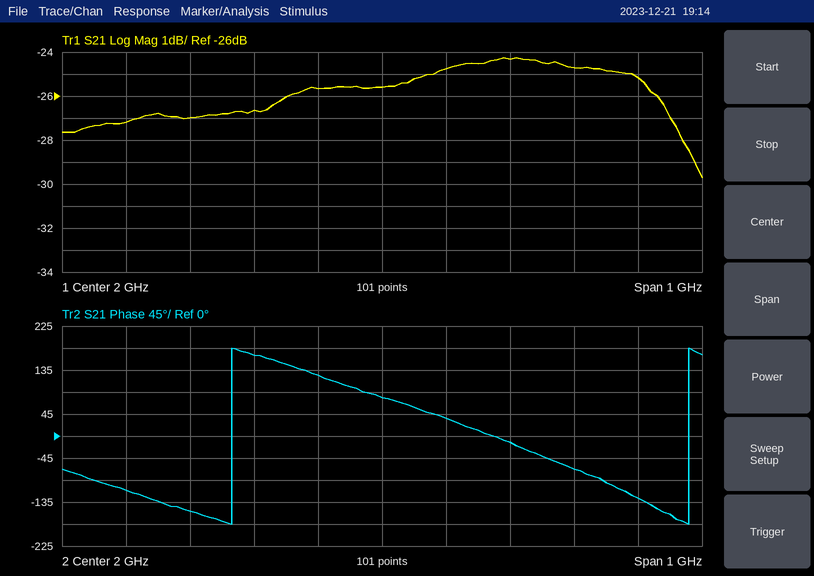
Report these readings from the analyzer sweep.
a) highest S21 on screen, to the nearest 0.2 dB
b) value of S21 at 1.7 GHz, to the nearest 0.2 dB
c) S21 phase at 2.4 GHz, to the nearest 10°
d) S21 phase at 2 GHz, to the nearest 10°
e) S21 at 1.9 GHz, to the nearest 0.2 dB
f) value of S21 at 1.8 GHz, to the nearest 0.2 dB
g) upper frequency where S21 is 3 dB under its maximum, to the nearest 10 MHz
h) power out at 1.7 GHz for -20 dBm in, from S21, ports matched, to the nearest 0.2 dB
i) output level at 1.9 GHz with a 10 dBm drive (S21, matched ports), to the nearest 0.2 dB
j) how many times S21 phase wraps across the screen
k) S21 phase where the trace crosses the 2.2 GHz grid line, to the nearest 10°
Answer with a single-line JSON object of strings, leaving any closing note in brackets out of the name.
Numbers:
{"highest S21 on screen, to the nearest 0.2 dB": "-24.2 dB", "value of S21 at 1.7 GHz, to the nearest 0.2 dB": "-27.0 dB", "S21 phase at 2.4 GHz, to the nearest 10°": "-130°", "S21 phase at 2 GHz, to the nearest 10°": "80°", "S21 at 1.9 GHz, to the nearest 0.2 dB": "-25.6 dB", "value of S21 at 1.8 GHz, to the nearest 0.2 dB": "-26.6 dB", "upper frequency where S21 is 3 dB under its maximum, to the nearest 10 MHz": "2.46 GHz", "power out at 1.7 GHz for -20 dBm in, from S21, ports matched, to the nearest 0.2 dB": "-47.0 dBm", "output level at 1.9 GHz with a 10 dBm drive (S21, matched ports), to the nearest 0.2 dB": "-15.6 dBm", "how many times S21 phase wraps across the screen": "2", "S21 phase where the trace crosses the 2.2 GHz grid line, to the nearest 10°": "-10°"}
